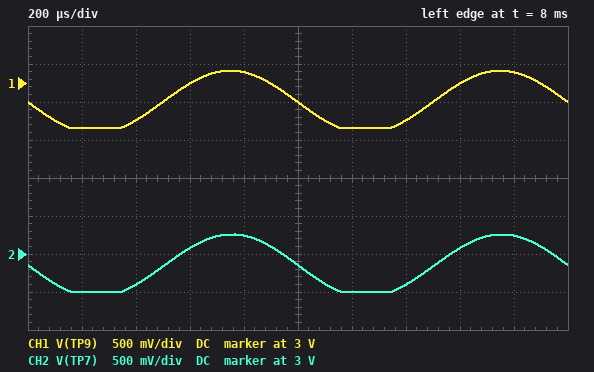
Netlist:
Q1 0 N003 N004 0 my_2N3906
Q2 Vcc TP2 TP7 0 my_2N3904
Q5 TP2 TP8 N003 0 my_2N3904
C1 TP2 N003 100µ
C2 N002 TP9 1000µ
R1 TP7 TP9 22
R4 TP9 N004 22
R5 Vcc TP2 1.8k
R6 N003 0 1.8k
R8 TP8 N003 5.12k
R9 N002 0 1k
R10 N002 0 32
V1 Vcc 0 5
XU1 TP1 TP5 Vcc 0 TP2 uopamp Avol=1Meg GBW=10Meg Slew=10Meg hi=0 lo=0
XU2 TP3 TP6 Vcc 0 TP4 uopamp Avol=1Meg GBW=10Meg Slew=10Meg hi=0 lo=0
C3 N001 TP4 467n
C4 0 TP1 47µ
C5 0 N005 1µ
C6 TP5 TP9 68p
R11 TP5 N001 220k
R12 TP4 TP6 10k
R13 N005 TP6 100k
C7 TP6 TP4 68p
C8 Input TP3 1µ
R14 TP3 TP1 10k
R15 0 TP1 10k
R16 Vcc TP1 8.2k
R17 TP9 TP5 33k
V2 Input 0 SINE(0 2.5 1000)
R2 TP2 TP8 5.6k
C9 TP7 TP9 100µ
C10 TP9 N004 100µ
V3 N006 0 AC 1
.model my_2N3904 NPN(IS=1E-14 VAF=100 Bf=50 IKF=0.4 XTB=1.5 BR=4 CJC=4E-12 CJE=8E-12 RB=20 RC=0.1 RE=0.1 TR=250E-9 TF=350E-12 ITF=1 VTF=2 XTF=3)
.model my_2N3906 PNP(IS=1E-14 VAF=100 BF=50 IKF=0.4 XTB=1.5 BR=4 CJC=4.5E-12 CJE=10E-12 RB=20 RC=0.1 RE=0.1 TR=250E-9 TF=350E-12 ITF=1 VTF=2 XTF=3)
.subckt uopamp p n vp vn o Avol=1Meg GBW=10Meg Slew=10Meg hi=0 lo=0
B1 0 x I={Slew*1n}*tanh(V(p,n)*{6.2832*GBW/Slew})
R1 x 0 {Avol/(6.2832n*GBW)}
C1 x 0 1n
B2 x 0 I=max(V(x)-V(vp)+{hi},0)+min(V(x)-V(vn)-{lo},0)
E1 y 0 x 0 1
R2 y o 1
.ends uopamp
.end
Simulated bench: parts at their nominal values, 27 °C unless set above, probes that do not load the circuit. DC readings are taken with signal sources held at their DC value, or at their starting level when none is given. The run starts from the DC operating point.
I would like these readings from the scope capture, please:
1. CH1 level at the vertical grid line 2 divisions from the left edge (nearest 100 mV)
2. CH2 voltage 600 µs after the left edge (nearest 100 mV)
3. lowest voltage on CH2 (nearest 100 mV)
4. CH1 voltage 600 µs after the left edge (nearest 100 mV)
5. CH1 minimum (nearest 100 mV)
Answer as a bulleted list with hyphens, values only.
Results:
- 2.5 V
- 3.1 V
- 2.5 V
- 3.0 V
- 2.4 V
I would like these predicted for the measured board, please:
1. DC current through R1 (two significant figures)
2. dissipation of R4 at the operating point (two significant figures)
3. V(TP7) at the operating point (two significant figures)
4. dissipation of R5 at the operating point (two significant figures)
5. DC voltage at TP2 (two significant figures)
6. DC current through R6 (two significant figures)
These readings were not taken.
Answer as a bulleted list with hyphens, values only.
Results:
- 2.5 mA
- 140 µW
- 2.8 V
- 1.3 mW
- 3.5 V
- 1.1 mA
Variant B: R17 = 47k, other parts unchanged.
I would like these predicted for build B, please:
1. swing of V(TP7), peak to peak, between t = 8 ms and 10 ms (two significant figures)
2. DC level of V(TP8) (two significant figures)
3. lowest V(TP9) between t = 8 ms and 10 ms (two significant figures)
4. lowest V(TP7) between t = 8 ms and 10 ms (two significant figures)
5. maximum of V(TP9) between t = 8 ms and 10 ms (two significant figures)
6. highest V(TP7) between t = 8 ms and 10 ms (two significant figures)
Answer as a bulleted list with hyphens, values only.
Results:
- 1.1 V
- 2.7 V
- 2.3 V
- 2.4 V
- 3.3 V
- 3.5 V
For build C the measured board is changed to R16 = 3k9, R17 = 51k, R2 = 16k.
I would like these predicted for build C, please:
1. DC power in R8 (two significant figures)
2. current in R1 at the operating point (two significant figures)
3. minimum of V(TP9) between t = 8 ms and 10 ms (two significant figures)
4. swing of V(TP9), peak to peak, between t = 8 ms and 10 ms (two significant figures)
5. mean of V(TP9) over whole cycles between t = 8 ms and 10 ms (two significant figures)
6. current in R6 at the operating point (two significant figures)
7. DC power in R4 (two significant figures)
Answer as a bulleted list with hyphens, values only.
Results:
- 79 µW
- 29 mA
- 3.3 V
- 390 mV
- 3.5 V
- 1.2 mA
- 18 mW
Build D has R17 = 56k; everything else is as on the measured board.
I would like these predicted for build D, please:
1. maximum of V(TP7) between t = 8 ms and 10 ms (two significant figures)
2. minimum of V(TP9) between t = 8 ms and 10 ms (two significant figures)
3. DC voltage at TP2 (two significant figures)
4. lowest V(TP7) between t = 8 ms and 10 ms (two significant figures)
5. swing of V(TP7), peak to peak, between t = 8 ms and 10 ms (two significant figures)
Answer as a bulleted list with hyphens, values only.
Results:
- 3.6 V
- 2.2 V
- 3.5 V
- 2.3 V
- 1.3 V
